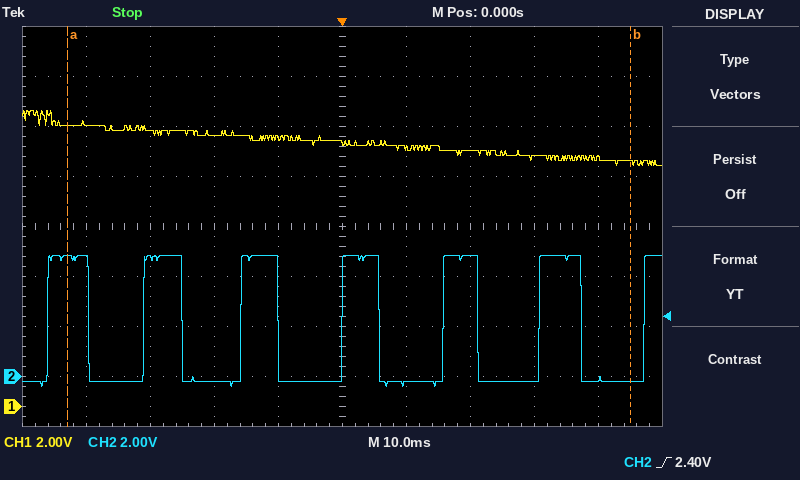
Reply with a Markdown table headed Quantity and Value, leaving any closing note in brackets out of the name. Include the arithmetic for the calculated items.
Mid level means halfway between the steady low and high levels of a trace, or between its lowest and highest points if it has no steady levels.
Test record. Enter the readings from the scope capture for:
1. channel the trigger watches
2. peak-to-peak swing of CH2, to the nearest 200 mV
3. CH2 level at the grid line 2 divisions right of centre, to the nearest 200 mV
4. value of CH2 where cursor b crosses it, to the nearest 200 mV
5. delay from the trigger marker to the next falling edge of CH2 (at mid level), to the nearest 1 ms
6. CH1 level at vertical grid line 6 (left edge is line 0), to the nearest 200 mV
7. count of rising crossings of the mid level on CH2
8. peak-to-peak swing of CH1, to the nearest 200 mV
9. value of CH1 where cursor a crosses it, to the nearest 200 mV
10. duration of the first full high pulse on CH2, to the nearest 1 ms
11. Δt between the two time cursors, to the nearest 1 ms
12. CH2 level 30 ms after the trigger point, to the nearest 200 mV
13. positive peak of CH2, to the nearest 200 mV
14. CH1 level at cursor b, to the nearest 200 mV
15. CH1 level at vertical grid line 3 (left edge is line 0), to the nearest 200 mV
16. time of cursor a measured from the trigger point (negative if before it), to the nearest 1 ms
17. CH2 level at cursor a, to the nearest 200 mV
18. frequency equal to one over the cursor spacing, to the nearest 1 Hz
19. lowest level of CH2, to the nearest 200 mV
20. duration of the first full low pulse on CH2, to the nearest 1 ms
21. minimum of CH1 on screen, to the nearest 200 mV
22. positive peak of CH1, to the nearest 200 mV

| Quantity | Value |
|---|---|
| channel the trigger watches | CH2 |
| peak-to-peak swing of CH2, to the nearest 200 mV | 4.8 V − (-400 mV) = 5.2 V |
| CH2 level at the grid line 2 divisions right of centre, to the nearest 200 mV | 4.8 V |
| value of CH2 where cursor b crosses it, to the nearest 200 mV | -200 mV |
| delay from the trigger marker to the next falling edge of CH2 (at mid level), to the nearest 1 ms | 6 ms |
| CH1 level at vertical grid line 6 (left edge is line 0), to the nearest 200 mV | 10.4 V |
| count of rising crossings of the mid level on CH2 | 7 |
| peak-to-peak swing of CH1, to the nearest 200 mV | 11.8 V − (9.6 V) = 2.2 V |
| value of CH1 where cursor a crosses it, to the nearest 200 mV | 11.2 V |
| duration of the first full high pulse on CH2, to the nearest 1 ms | 6 ms |
| Δt between the two time cursors, to the nearest 1 ms | 88 ms |
| CH2 level 30 ms after the trigger point, to the nearest 200 mV | -200 mV |
| positive peak of CH2, to the nearest 200 mV | 4.8 V |
| CH1 level at cursor b, to the nearest 200 mV | 9.8 V |
| CH1 level at vertical grid line 3 (left edge is line 0), to the nearest 200 mV | 10.8 V |
| time of cursor a measured from the trigger point (negative if before it), to the nearest 1 ms | -43 ms |
| CH2 level at cursor a, to the nearest 200 mV | 4.8 V |
| frequency equal to one over the cursor spacing, to the nearest 1 Hz | 1 / 88 ms ≈ 11 Hz |
| lowest level of CH2, to the nearest 200 mV | -400 mV |
| duration of the first full low pulse on CH2, to the nearest 1 ms | 9 ms |
| minimum of CH1 on screen, to the nearest 200 mV | 9.6 V |
| positive peak of CH1, to the nearest 200 mV | 11.8 V |
